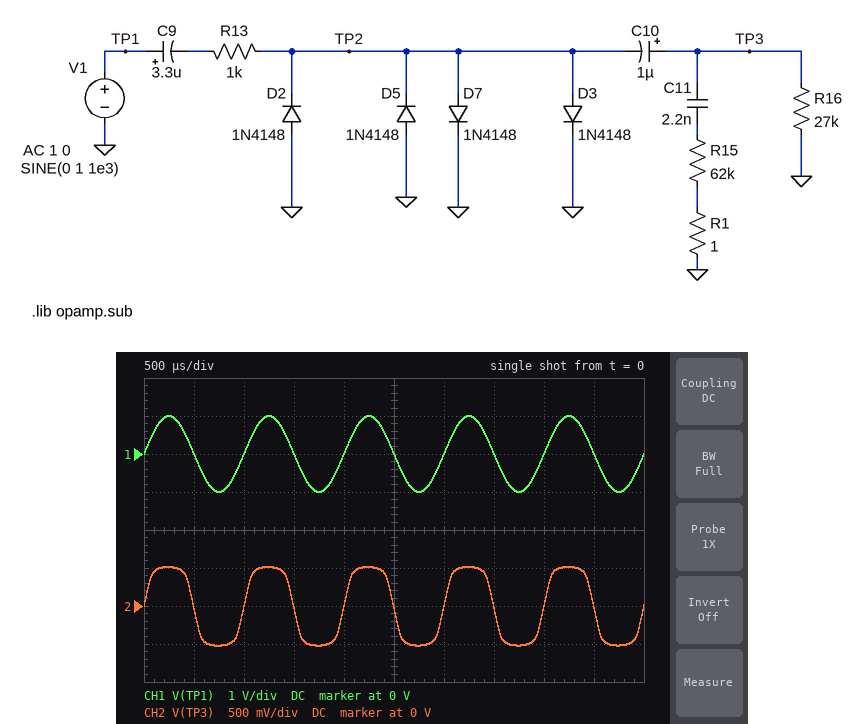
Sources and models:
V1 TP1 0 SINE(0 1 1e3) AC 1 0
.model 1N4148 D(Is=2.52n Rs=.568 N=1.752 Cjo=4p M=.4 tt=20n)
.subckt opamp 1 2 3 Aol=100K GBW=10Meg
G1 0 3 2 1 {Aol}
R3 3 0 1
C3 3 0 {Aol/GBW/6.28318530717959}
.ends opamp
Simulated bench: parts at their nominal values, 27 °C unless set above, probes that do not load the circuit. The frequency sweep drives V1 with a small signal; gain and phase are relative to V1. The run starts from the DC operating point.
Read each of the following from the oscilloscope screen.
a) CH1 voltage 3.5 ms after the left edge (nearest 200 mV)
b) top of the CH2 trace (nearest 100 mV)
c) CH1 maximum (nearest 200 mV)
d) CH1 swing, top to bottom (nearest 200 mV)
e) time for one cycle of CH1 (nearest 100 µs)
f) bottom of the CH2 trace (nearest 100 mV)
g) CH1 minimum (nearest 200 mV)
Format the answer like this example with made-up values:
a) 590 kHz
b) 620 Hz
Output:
a) 0 V
b) 500 mV
c) 1.0 V
d) 2.0 V
e) 1.0 ms
f) -500 mV
g) -1.0 V
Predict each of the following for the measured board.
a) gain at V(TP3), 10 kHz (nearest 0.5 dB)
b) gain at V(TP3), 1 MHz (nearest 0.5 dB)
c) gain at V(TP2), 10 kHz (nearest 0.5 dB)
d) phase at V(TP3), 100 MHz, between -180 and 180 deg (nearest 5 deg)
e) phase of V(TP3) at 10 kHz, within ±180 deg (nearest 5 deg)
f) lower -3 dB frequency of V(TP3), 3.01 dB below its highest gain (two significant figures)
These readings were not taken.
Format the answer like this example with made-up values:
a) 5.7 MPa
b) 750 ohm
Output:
a) -0.5 dB
b) -0.5 dB
c) -0.5 dB
d) -85 deg
e) 0 deg
f) 7.4 Hz
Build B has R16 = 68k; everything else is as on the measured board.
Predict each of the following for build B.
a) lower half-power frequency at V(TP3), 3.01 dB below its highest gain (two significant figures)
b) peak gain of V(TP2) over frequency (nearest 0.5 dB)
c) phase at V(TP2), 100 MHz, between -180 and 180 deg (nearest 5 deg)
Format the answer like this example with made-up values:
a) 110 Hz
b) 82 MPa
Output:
a) 3.0 Hz
b) 0 dB
c) -85 deg
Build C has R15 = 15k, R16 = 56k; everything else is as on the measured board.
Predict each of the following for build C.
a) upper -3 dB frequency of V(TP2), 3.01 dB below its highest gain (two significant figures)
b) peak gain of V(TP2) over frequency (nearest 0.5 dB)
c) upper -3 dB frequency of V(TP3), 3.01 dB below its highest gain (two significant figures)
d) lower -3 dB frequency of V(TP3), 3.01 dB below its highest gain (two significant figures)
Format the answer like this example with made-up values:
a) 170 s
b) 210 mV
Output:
a) 9.4 MHz
b) 0 dB
c) 9.5 MHz
d) 3.6 Hz
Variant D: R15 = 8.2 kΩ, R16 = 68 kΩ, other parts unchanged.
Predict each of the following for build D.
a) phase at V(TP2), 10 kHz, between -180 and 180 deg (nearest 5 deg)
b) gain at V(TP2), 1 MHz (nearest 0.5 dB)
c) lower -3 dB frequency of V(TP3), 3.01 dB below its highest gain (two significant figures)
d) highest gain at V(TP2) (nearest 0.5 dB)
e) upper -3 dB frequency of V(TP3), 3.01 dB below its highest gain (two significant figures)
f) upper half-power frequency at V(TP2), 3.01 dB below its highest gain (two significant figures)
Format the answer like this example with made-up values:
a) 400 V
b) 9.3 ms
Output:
a) -5 deg
b) -1.0 dB
c) 3.0 Hz
d) 0 dB
e) 8.8 MHz
f) 8.7 MHz
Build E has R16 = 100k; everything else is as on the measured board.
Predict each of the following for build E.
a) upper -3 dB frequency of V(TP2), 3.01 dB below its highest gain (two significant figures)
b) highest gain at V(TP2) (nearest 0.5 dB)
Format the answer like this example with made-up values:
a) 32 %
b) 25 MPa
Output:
a) 9.9 MHz
b) 0 dB
